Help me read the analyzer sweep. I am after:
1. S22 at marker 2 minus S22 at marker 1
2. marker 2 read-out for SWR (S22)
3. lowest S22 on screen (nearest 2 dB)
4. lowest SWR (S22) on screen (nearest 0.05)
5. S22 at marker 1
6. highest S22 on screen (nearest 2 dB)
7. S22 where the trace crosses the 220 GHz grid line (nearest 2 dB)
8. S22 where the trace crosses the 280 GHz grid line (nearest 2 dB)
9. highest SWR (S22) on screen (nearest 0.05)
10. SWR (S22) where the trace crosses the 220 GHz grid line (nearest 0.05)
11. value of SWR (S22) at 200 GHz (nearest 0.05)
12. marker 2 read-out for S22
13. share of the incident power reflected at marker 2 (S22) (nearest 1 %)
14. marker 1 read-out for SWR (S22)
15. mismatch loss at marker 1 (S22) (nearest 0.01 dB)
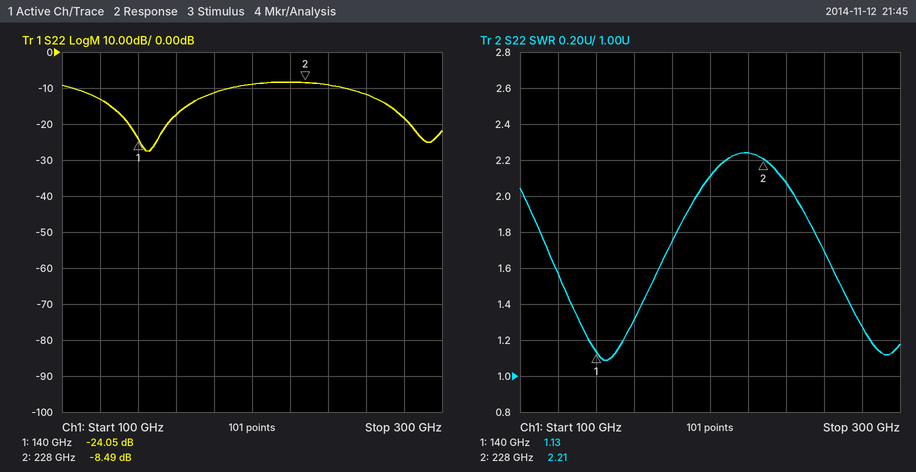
15.56 dB
2.21
-28 dB
1.10
-24.05 dB
-8 dB
-8 dB
-18 dB
2.25
2.25
2.10
-8.49 dB
14 %
1.13
0.02 dB
